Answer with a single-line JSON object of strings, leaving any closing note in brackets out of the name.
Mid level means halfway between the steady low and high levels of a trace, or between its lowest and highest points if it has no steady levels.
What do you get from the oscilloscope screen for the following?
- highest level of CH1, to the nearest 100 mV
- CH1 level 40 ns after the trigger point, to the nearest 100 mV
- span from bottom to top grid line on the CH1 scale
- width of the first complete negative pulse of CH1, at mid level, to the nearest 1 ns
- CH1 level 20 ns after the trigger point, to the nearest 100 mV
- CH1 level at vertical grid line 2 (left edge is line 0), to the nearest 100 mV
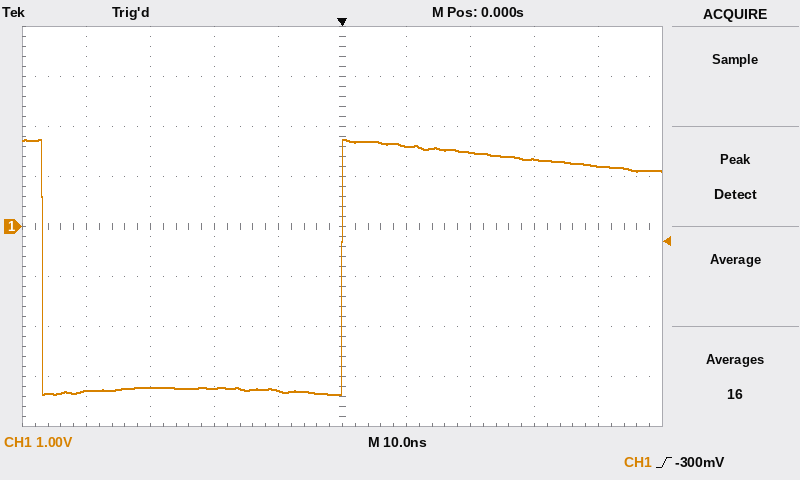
{"highest level of CH1, to the nearest 100 mV": "1.7 V", "CH1 level 40 ns after the trigger point, to the nearest 100 mV": "1.2 V", "span from bottom to top grid line on the CH1 scale": "8 V", "width of the first complete negative pulse of CH1, at mid level, to the nearest 1 ns": "47 ns", "CH1 level 20 ns after the trigger point, to the nearest 100 mV": "1.5 V", "CH1 level at vertical grid line 2 (left edge is line 0), to the nearest 100 mV": "-3.2 V"}
